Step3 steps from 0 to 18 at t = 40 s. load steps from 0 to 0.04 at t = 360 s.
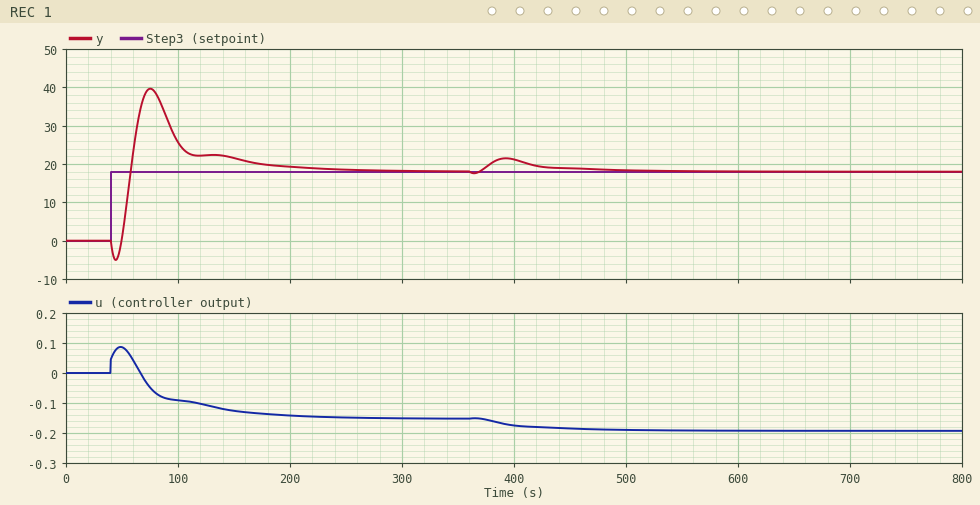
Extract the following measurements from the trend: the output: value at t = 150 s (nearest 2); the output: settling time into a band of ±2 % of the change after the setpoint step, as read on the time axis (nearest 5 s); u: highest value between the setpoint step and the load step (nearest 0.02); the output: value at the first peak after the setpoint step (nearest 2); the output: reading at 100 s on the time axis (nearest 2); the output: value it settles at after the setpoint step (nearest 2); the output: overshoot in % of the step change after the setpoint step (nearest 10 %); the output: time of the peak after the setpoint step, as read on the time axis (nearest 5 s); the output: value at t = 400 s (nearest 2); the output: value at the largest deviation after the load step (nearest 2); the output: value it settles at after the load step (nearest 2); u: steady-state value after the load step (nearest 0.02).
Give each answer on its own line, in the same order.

22
270 s
0.08
40
26
18
120 %
75 s
22
22
18
-0.20
